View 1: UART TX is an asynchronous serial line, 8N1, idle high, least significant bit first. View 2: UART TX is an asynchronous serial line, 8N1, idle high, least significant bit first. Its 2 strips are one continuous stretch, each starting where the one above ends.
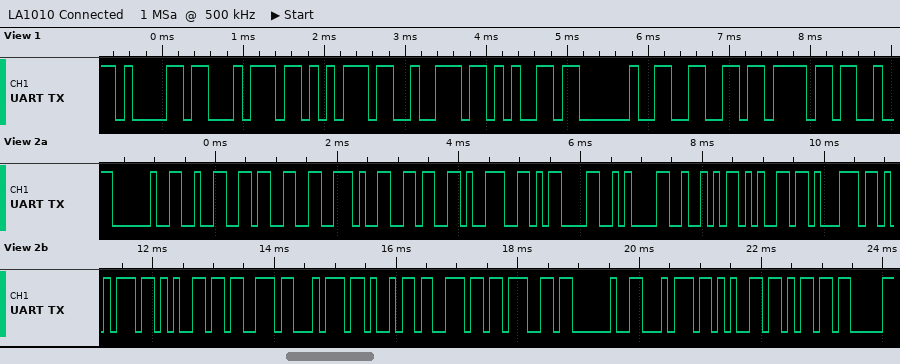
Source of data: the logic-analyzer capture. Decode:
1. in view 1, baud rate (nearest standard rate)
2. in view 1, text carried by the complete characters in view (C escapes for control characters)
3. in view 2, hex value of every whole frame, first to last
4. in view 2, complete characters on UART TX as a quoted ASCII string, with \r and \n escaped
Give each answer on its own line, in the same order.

9600 baud
"ature fo"
0x20 0x32 0x33 0x2E 0x36 0x39 0x0D 0x0A 0x52 0x65 0x71 0x75 0x65 0x73 0x74 0x69 0x6E 0x67 0x20 0x74 0x65 0x6D
" 23.69\r\nRequesting tem"
